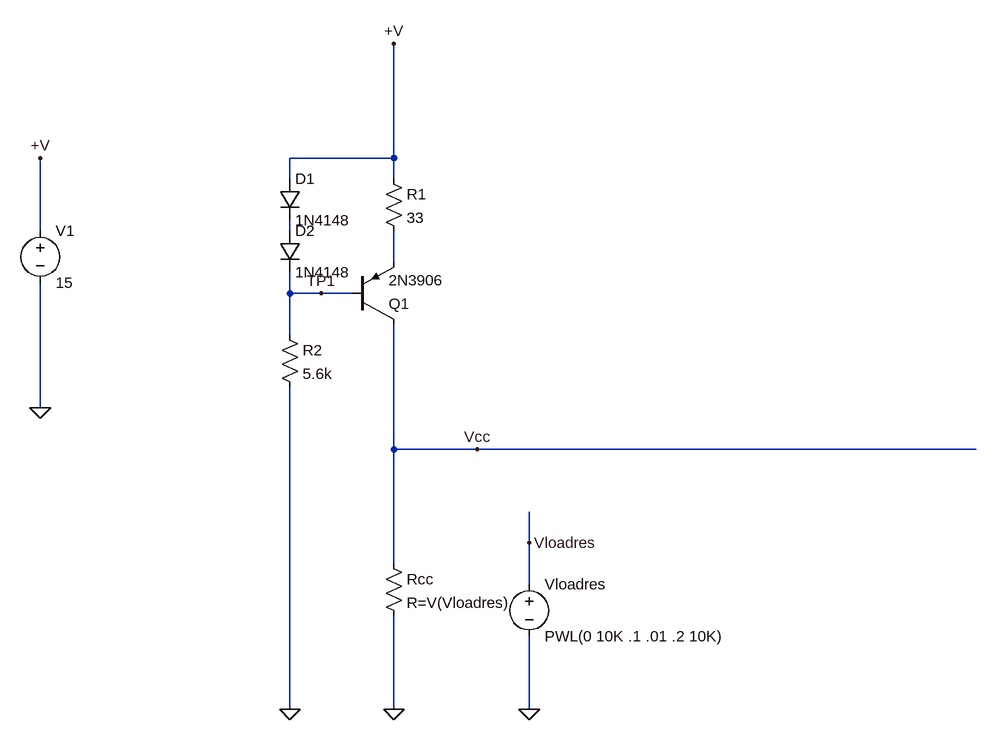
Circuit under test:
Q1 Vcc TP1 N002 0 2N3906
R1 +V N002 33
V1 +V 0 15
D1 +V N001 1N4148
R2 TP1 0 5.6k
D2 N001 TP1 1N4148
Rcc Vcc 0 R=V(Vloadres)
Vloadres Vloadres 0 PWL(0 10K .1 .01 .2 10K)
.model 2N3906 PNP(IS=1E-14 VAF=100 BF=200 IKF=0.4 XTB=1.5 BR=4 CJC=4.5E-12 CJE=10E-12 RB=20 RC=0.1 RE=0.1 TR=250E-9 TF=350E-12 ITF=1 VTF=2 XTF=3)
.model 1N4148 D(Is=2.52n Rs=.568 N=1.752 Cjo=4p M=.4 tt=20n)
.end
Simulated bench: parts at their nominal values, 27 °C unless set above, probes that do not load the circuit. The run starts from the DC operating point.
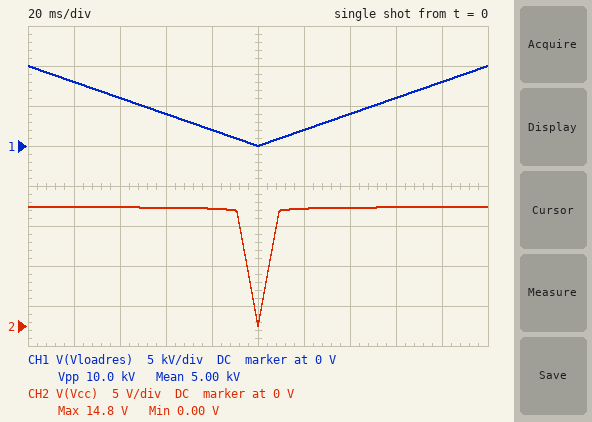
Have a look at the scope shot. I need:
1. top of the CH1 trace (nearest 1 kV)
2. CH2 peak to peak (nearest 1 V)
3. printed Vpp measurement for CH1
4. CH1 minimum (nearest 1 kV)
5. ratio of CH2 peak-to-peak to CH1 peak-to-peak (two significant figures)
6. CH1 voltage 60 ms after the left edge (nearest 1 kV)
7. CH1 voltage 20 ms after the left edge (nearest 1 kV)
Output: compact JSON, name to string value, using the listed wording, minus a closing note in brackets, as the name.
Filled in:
{"top of the CH1 trace": "10 kV", "CH2 peak to peak": "15 V", "printed Vpp measurement for CH1": "10.0 kV", "CH1 minimum": "0 V", "ratio of CH2 peak-to-peak to CH1 peak-to-peak": "0.0015", "CH1 voltage 60 ms after the left edge": "4 kV", "CH1 voltage 20 ms after the left edge": "8 kV"}
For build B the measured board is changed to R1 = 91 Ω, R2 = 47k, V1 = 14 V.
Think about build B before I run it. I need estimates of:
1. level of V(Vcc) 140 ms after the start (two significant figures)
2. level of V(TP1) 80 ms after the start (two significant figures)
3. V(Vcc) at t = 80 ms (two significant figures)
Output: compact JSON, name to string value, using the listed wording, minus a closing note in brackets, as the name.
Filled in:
{"level of V(Vcc) 140 ms after the start": "14 V", "level of V(TP1) 80 ms after the start": "13 V", "V(Vcc) at t = 80 ms": "7.8 V"}
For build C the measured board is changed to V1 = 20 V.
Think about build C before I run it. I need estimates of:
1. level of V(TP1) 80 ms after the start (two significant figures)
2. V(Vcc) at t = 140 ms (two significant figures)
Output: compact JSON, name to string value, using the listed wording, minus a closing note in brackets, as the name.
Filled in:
{"level of V(TP1) 80 ms after the start": "19 V", "V(Vcc) at t = 140 ms": "20 V"}
